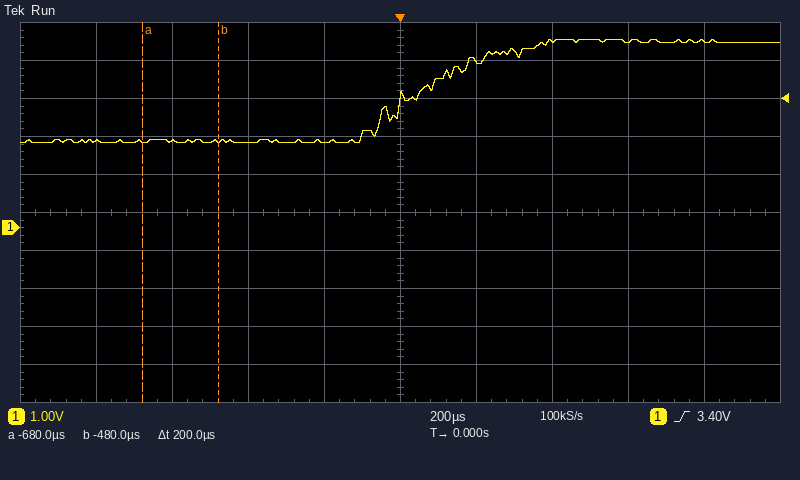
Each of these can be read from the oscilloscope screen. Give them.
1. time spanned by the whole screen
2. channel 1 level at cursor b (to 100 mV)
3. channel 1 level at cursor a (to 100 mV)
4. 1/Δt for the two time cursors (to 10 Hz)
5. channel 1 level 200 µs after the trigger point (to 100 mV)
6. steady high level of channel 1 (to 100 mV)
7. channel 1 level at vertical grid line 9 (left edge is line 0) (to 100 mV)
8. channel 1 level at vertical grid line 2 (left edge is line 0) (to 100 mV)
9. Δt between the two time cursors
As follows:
2 ms
2.3 V
2.3 V
5.00 kHz
4.4 V
4.9 V
4.9 V
2.3 V
200 µs
